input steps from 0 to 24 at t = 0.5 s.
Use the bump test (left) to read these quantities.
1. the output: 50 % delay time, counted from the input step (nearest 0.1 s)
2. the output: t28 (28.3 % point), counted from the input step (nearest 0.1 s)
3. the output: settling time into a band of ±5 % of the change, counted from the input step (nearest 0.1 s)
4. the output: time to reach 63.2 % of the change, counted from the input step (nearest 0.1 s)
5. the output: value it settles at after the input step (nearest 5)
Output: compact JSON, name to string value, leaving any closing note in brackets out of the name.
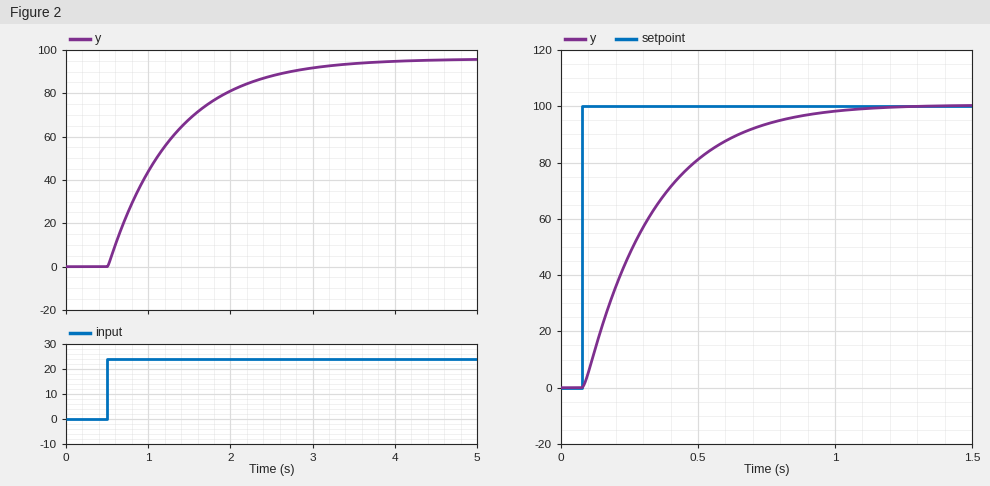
{"the output: 50 % delay time, counted from the input step": "0.6 s", "the output: t28 (28.3 % point), counted from the input step": "0.3 s", "the output: settling time into a band of ±5 % of the change, counted from the input step": "2.4 s", "the output: time to reach 63.2 % of the change, counted from the input step": "0.8 s", "the output: value it settles at after the input step": "95"}
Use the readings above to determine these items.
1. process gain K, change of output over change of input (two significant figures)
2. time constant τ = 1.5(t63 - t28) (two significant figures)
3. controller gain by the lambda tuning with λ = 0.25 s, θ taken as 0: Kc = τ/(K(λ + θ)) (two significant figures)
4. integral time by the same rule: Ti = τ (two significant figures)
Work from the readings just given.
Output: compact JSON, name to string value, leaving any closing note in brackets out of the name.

{"process gain K, change of output over change of input": "4.0", "time constant τ = 1.5(t63 - t28)": "0.75 s", "controller gain by the lambda tuning with λ = 0.25 s, θ taken as 0: Kc = τ/(K(λ + θ))": "0.75", "integral time by the same rule: Ti = τ": "0.75 s"}
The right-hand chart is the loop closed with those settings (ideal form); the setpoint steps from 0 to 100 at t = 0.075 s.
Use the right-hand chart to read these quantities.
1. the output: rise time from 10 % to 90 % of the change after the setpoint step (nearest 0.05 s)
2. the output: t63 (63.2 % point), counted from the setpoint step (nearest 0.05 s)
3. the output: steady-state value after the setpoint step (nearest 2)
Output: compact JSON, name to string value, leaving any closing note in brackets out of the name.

{"the output: rise time from 10 % to 90 % of the change after the setpoint step": "0.55 s", "the output: t63 (63.2 % point), counted from the setpoint step": "0.25 s", "the output: steady-state value after the setpoint step": "100"}
